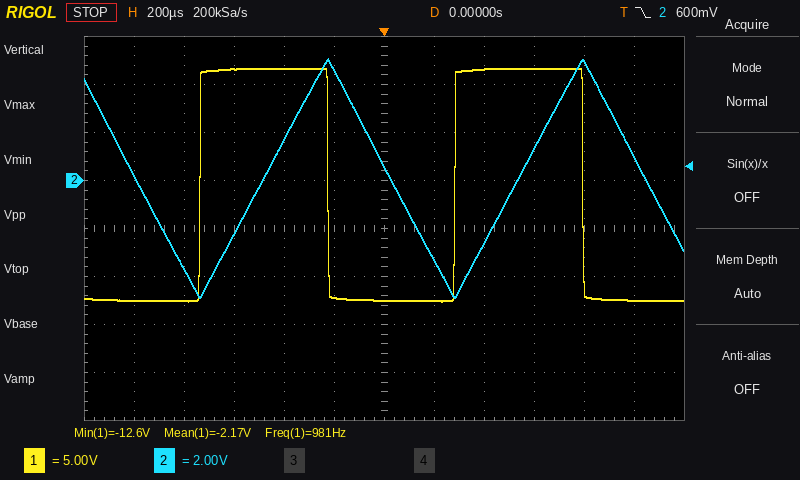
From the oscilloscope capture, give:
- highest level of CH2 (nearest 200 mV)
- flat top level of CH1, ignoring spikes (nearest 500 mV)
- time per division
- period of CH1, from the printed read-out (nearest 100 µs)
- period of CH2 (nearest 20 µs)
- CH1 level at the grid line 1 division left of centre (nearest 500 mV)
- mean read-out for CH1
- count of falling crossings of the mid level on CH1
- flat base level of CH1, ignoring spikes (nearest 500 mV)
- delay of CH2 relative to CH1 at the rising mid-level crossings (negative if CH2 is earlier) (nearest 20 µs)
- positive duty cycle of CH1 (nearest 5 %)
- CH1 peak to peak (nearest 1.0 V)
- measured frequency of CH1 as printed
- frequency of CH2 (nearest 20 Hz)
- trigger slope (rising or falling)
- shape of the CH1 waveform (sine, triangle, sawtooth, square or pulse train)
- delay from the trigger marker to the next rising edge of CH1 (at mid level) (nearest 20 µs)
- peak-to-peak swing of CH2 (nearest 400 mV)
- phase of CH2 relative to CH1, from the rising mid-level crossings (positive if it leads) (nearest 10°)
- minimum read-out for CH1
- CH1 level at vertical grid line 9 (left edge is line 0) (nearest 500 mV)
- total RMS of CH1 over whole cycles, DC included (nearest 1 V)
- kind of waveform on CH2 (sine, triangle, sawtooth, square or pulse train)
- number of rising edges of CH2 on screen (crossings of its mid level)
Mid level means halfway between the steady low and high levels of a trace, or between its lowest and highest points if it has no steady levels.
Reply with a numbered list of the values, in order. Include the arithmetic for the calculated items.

1. 5.0 V
2. 11.5 V
3. 200 µs
4. 1 / 981 Hz ≈ 1.0 ms
5. 1.02 ms
6. -12.0 V
7. -2.17 V
8. 2
9. -12.5 V
10. +260 µs
11. 50 %
12. 24.0 V
13. 981 Hz
14. 1 / 1.02 ms ≈ 980 Hz
15. falling
16. square
17. 280 µs
18. 10.0 V
19. −360° × (+260 µs) / 1.02 ms ≈ -91.8°, so -90° to the nearest 10°
20. -12.6 V
21. 11.5 V
22. √(0.5 × (11.5 V)² + 0.5 × (-12.5 V)²) ≈ 12 V
23. triangle
24. 2
